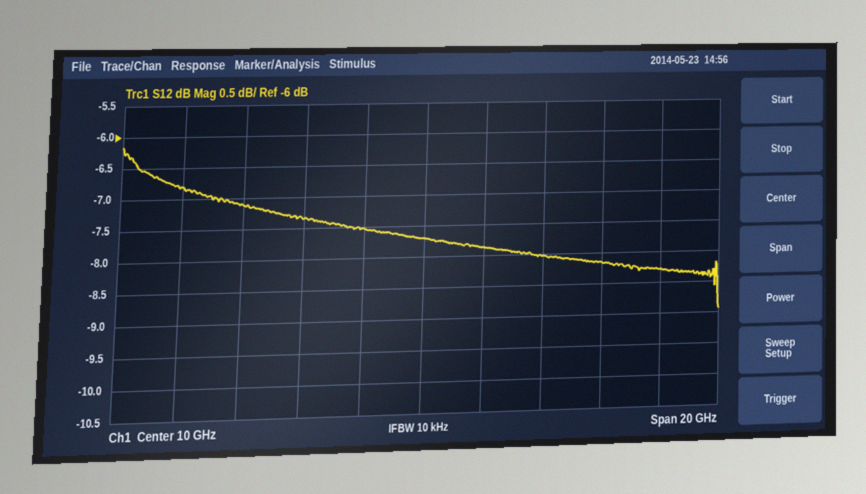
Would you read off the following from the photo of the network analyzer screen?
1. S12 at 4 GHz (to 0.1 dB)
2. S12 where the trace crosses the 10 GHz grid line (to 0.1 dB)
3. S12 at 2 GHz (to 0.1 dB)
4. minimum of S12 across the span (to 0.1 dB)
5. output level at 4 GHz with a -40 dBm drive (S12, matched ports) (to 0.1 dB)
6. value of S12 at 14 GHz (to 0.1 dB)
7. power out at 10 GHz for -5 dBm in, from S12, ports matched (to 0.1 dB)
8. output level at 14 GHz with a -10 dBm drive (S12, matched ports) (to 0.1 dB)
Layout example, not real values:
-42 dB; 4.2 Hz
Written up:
-7.1 dB; -7.7 dB; -6.8 dB; -8.9 dB; -47.1 dBm; -8.0 dB; -12.7 dBm; -18.0 dBm
